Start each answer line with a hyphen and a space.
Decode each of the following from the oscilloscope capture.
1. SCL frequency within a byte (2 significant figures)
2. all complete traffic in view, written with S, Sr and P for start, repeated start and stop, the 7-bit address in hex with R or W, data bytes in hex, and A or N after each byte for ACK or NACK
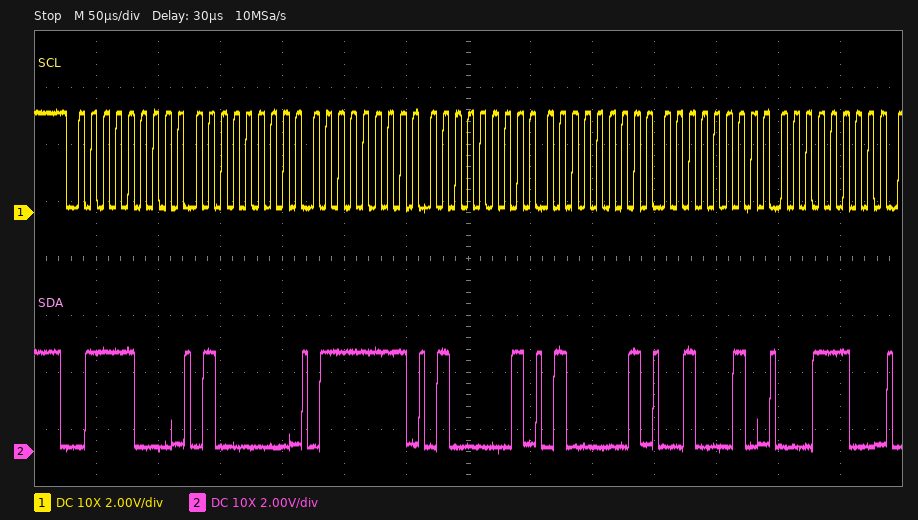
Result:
- 100 kHz
- S 3CW A 40 A 7F A 41 A 41 A 22 A 1C A
